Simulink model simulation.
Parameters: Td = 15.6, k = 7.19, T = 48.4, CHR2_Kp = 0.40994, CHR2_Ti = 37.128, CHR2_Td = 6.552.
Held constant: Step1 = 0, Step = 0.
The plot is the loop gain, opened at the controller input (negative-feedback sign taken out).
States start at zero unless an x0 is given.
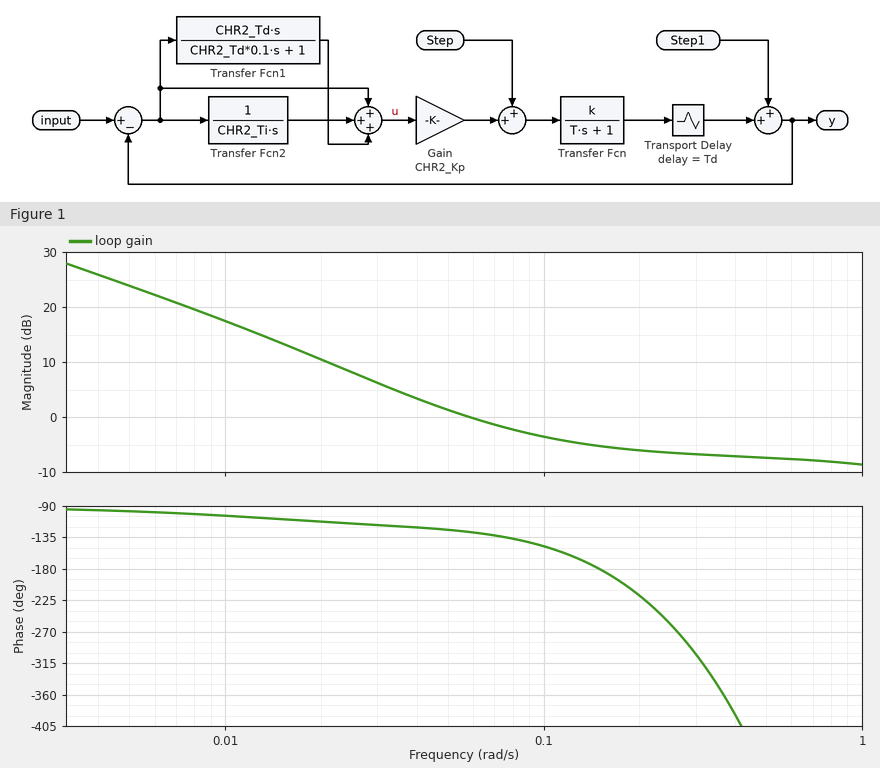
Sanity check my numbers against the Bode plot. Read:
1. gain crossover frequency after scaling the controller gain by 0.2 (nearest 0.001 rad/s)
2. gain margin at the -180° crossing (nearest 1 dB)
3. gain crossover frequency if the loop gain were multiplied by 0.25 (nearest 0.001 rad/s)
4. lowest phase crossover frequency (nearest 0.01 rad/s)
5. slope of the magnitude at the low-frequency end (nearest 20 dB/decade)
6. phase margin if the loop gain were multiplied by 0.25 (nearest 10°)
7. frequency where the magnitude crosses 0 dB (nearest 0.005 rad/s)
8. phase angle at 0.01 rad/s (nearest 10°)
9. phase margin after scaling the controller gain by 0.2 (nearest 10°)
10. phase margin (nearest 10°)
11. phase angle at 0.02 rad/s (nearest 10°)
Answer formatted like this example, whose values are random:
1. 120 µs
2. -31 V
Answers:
1. 0.014 rad/s
2. 5 dB
3. 0.017 rad/s
4. 0.15 rad/s
5. -20 dB/decade
6. 70°
7. 0.060 rad/s
8. -100°
9. 70°
10. 50°
11. -110°
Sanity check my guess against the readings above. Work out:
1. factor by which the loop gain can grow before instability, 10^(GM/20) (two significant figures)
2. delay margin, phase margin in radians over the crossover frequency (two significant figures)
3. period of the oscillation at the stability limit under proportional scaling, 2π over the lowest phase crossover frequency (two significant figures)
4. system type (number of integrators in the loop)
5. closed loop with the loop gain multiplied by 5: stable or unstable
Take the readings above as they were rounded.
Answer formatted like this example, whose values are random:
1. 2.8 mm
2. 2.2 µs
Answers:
1. 1.8
2. 15 s
3. 42 s
4. 1
5. unstable
